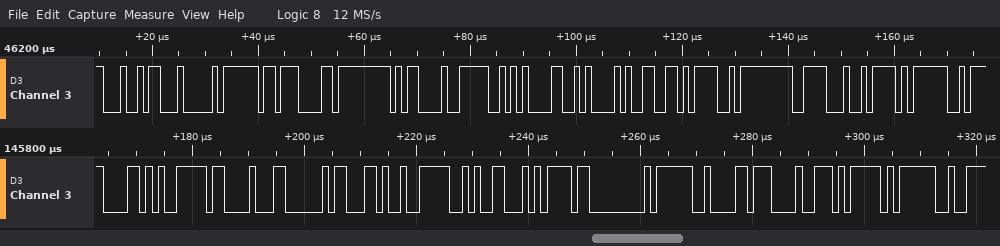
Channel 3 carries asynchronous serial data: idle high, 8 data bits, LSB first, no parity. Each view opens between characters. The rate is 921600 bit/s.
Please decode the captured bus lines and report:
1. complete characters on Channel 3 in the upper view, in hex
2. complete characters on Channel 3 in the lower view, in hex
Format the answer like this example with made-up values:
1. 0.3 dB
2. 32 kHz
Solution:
1. A4, 04, BF, 87, FF, 0D, 3E, 85, 0A, 99, 3D, FF, 1E, 7A, 3F
2. 58, BE, 88, A0, 2C, 3E, 19, BD, 00, 3F, D8, C8, 7D, 3F
